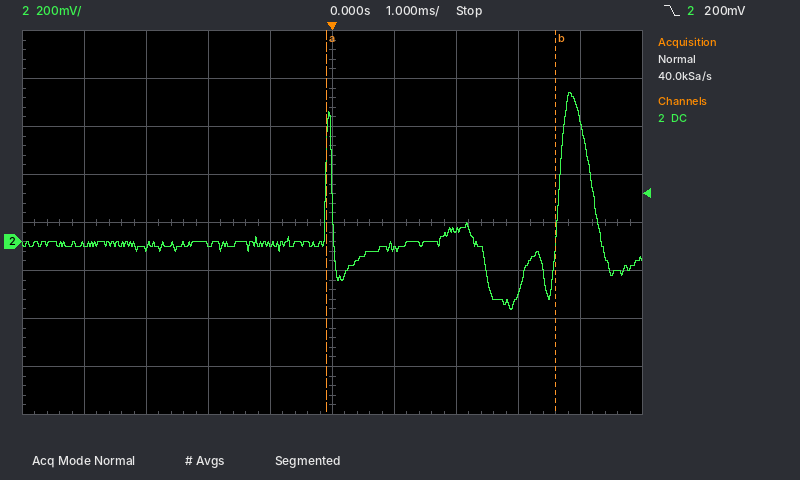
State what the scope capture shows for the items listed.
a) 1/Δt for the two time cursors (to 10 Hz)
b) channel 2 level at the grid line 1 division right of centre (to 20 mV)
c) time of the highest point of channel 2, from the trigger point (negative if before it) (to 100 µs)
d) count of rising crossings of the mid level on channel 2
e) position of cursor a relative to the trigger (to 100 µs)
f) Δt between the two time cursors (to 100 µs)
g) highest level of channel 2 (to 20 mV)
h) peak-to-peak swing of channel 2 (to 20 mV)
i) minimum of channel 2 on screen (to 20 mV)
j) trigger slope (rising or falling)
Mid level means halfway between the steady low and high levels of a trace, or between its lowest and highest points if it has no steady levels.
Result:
270 Hz
-20 mV
+3.8 ms
2
-100 µs
3.7 ms
620 mV
900 mV
-280 mV
falling
